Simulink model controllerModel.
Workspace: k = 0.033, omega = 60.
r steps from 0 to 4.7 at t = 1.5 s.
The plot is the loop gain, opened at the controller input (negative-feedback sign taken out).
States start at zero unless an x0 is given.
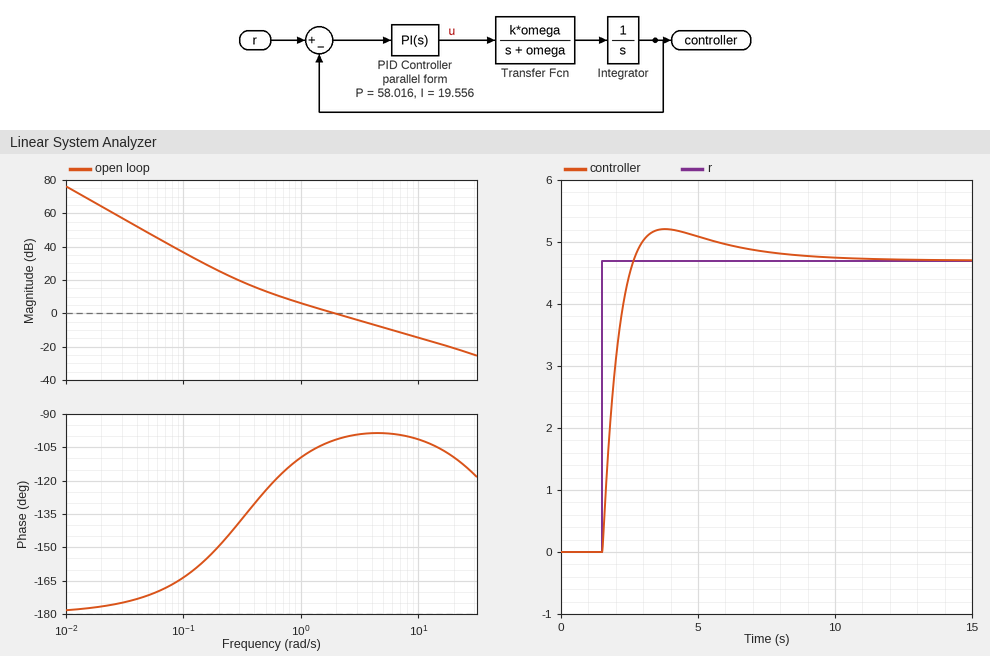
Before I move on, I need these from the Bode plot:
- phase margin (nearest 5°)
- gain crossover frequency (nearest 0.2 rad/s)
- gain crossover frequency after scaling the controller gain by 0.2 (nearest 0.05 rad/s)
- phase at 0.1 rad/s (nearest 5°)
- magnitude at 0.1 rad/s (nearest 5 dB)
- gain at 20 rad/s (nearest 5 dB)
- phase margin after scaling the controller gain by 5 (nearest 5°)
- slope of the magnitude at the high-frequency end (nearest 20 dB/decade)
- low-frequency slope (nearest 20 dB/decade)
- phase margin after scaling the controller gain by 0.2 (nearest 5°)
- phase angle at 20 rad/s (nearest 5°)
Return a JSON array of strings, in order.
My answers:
["80°", "2.0 rad/s", "0.45 rad/s", "-165°", "35 dB", "-20 dB", "80°", "-20 dB/decade", "-40 dB/decade", "55°", "-110°"]
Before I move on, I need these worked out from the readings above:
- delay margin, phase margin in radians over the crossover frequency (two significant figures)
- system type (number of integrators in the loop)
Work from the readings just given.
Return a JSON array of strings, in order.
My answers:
["0.70 s", "2"]
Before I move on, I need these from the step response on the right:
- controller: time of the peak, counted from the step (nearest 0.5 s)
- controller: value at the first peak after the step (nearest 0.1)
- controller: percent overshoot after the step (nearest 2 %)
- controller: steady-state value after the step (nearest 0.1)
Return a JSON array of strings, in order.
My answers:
["2.5 s", "5.2", "10 %", "4.7"]
